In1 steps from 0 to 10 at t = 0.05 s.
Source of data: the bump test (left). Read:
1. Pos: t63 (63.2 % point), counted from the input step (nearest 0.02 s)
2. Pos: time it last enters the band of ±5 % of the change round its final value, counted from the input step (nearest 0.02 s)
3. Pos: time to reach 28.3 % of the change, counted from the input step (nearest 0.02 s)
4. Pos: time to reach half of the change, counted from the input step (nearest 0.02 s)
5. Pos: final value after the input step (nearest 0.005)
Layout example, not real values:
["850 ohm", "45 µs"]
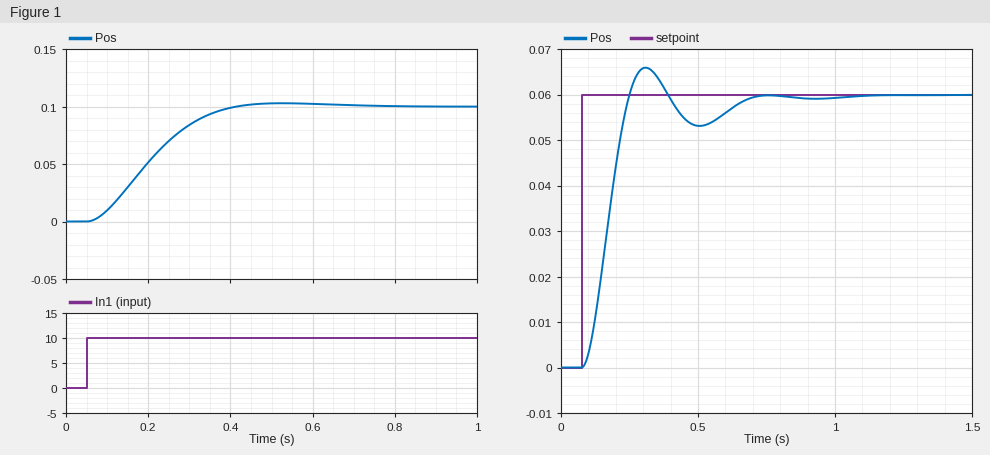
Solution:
["0.18 s", "0.32 s", "0.10 s", "0.14 s", "0.100"]
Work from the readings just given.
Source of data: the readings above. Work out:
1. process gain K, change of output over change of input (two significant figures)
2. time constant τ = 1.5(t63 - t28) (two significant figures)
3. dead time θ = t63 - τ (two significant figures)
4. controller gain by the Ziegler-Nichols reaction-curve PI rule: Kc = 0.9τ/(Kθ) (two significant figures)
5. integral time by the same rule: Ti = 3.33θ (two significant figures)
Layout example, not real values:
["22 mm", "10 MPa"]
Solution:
["0.010", "0.12 s", "0.060 s", "180", "0.20 s"]
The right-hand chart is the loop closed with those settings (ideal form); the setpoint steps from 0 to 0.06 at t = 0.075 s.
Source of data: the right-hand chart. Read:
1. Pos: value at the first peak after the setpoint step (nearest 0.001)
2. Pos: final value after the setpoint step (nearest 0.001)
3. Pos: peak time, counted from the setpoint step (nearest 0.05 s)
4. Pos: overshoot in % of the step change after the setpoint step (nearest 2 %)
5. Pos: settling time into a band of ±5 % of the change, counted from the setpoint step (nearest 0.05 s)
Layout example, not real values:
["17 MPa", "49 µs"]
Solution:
["0.066", "0.060", "0.25 s", "10 %", "0.55 s"]
